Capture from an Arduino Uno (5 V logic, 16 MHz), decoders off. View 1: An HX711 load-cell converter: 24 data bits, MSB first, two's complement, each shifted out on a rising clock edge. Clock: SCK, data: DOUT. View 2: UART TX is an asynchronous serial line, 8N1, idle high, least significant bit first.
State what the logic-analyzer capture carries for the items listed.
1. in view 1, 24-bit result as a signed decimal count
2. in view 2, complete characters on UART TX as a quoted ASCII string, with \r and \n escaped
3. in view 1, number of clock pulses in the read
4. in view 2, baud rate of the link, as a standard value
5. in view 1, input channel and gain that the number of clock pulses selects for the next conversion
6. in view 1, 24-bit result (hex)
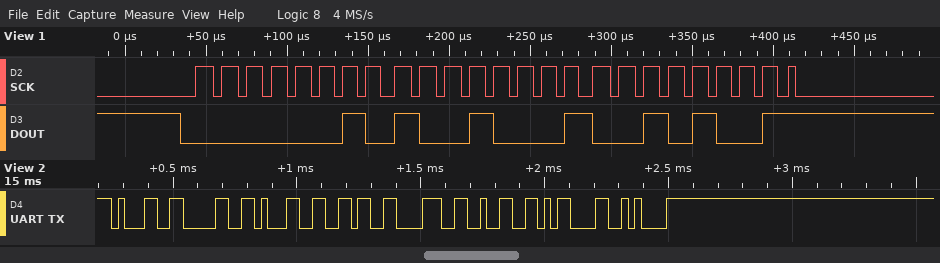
168233
"101682\r\n"
25
38400 baud
channel A, gain 128
0x029129
